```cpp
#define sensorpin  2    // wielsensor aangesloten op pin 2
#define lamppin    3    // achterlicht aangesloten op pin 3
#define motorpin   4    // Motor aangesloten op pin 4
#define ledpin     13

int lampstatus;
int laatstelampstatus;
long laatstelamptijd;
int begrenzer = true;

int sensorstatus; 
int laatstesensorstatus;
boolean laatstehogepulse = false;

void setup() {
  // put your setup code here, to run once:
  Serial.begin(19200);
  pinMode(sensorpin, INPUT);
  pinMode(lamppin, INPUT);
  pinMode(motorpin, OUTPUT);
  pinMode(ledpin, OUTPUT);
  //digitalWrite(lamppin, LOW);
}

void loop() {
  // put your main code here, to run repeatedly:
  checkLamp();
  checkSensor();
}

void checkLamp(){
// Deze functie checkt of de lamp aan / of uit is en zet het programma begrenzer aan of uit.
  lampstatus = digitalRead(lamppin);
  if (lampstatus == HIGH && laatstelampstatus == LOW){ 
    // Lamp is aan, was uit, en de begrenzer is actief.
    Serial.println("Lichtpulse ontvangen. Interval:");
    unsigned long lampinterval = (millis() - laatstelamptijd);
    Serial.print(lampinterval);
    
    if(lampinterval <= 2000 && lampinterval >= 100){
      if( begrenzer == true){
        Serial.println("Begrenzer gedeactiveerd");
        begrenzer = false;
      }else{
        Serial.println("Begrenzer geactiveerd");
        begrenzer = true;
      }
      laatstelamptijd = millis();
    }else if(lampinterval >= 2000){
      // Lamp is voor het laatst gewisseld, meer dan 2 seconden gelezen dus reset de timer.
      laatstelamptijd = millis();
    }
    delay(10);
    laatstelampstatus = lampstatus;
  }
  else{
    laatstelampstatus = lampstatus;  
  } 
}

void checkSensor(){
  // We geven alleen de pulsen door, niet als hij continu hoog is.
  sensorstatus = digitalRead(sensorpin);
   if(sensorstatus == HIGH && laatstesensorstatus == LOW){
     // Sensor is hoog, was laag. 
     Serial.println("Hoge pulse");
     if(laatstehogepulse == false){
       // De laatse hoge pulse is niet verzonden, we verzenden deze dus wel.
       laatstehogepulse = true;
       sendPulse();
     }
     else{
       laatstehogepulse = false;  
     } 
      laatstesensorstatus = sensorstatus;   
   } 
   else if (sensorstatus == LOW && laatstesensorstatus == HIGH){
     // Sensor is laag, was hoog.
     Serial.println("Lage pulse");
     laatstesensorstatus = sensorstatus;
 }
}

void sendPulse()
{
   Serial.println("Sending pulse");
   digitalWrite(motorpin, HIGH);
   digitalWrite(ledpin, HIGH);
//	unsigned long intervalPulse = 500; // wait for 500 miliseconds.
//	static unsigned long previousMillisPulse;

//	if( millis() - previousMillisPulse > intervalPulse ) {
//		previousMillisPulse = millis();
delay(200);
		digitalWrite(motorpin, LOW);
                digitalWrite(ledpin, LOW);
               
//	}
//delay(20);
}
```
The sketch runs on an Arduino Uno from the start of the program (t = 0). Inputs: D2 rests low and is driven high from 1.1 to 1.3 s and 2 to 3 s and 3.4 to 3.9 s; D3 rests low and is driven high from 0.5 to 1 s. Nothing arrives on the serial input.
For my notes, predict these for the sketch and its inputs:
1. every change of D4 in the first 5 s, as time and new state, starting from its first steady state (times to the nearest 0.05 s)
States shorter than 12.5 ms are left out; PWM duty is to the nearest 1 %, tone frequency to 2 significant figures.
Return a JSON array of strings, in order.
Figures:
["0 s low; 1.1 s high; 1.3 s low; 3.4 s high; 3.6 s low"]
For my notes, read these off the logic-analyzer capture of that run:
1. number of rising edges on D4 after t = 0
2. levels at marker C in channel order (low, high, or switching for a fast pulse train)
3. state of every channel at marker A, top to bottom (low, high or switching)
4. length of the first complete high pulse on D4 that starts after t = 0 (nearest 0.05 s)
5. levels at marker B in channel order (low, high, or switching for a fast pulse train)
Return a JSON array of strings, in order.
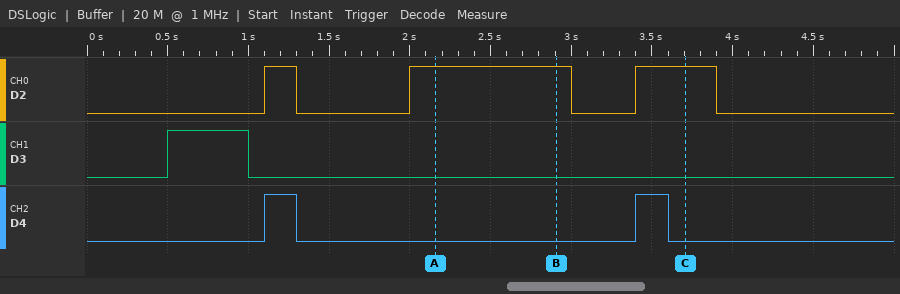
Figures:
["2", "D2 high, D3 low, D4 low", "D2 high, D3 low, D4 low", "0.20 s", "D2 high, D3 low, D4 low"]
